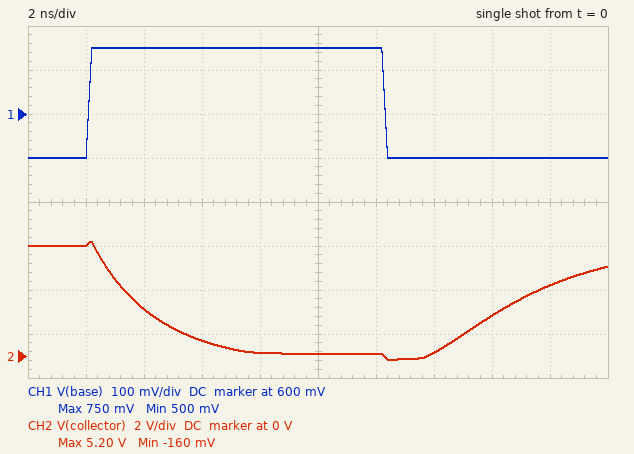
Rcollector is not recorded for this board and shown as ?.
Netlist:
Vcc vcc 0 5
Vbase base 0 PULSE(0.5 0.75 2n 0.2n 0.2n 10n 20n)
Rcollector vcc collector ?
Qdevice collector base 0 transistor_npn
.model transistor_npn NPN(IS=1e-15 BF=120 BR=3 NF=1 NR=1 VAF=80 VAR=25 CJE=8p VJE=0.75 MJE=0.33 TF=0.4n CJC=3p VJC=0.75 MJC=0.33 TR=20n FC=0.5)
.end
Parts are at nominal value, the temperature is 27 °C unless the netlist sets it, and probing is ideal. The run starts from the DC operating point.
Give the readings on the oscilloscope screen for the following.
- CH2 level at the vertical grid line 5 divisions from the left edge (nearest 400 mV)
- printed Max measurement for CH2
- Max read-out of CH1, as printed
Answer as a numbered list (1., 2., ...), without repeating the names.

1. 0 V
2. 5.20 V
3. 750 mV
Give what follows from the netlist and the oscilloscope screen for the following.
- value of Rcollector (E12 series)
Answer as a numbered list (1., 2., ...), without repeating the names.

1. 1.8 kΩ
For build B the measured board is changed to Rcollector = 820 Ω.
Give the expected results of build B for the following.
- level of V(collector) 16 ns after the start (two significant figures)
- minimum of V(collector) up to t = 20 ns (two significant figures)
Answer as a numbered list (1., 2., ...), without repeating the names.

1. 4.8 V
2. 1.8 V
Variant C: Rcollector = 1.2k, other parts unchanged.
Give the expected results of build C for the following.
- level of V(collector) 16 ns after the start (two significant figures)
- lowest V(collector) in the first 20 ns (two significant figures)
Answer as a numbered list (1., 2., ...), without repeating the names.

1. 4.0 V
2. 560 mV
